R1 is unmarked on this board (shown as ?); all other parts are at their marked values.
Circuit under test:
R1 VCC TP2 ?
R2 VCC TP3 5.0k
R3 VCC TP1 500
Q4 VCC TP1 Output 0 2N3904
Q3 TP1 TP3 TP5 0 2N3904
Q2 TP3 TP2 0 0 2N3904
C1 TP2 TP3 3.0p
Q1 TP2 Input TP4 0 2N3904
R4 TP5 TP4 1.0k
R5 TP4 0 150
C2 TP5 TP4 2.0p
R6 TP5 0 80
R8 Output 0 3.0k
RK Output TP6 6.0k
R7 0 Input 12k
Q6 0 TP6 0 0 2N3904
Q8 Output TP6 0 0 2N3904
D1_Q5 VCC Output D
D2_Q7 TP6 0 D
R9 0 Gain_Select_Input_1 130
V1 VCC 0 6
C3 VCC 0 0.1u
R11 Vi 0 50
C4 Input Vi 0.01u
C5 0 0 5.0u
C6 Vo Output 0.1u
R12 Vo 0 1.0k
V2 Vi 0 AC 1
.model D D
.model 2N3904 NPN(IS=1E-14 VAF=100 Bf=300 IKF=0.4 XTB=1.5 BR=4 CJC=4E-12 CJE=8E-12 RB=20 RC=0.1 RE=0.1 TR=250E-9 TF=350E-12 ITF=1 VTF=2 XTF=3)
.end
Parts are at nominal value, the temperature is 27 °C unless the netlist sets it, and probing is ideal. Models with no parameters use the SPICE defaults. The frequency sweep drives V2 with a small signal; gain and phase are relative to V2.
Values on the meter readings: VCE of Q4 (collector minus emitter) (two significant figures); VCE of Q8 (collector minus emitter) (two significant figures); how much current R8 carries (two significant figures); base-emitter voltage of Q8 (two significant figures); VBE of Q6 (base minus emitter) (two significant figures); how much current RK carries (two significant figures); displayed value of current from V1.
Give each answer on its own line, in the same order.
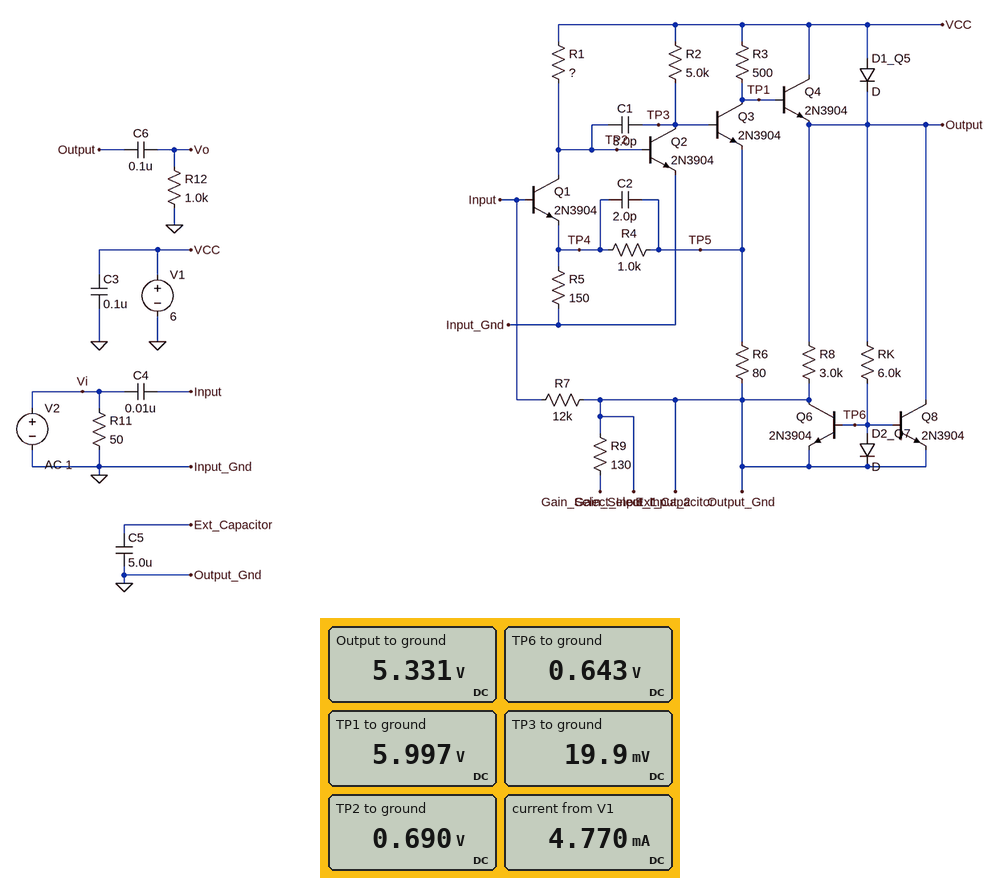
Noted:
670 mV
5.3 V
1.8 mA
640 mV
640 mV
780 µA
4.770 mA
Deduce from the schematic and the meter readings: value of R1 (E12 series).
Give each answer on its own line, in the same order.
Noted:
15 kΩ
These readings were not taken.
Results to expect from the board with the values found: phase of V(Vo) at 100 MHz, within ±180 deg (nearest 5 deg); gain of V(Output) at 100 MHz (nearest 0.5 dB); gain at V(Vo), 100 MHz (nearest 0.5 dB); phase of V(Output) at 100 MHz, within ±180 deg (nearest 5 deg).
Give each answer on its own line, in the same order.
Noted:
105 deg
-64.0 dB
-64.0 dB
105 deg
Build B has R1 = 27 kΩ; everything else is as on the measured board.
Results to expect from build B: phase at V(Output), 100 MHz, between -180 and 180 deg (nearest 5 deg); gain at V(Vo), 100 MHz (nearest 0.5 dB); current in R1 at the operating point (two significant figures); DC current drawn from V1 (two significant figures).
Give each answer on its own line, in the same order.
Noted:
100 deg
-61.5 dB
200 µA
4.6 mA
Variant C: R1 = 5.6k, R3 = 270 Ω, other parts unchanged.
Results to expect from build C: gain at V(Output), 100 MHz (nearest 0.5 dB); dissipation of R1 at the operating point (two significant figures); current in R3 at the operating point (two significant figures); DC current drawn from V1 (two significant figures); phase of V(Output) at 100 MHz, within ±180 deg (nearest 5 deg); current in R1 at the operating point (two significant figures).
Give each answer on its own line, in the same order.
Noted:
-68.5 dB
5.0 mW
5.2 µA
5.4 mA
125 deg
940 µA
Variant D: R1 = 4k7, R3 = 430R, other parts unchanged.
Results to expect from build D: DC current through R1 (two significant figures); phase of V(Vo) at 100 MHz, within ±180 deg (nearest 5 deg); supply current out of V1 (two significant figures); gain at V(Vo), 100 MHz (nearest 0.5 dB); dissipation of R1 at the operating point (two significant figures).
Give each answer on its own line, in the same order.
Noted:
1.1 mA
125 deg
5.5 mA
-69.0 dB
5.9 mW
